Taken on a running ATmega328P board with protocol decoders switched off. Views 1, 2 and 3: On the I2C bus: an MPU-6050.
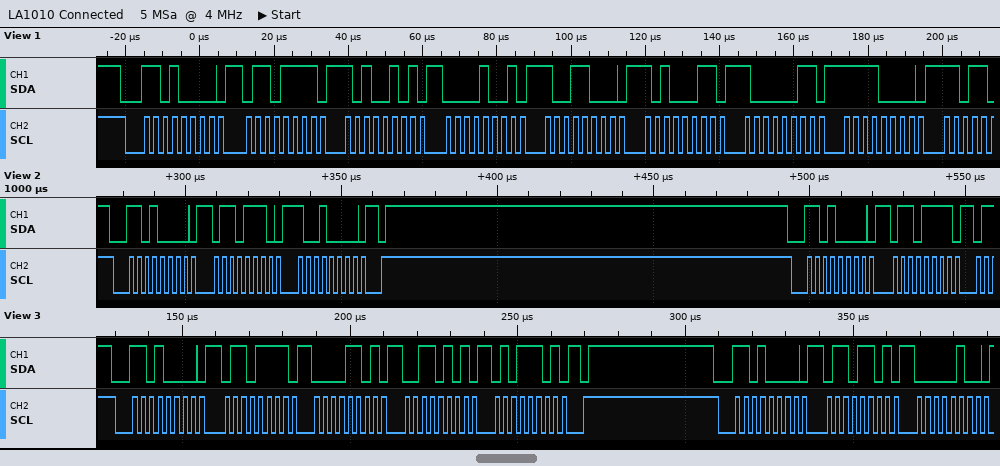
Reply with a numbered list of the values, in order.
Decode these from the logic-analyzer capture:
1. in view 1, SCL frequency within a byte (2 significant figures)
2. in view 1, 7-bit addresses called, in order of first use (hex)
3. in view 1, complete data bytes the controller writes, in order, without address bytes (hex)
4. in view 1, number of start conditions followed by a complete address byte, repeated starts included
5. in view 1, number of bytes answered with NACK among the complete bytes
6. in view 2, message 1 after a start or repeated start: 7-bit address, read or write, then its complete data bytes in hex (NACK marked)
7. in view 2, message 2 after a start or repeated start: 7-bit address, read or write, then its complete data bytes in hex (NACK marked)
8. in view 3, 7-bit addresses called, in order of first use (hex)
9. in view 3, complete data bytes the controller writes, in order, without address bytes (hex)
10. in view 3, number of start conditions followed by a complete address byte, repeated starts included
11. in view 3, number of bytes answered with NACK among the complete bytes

1. 400 kHz
2. 0x68
3. 6F A5 09 98 A3 83 F0
4. 1
5. 0
6. 0x68 write: 6E 90
7. 0x68 write: 6F
8. 0x68
9. 6F 0D 35 5D 6D 04
10. 2
11. 0
